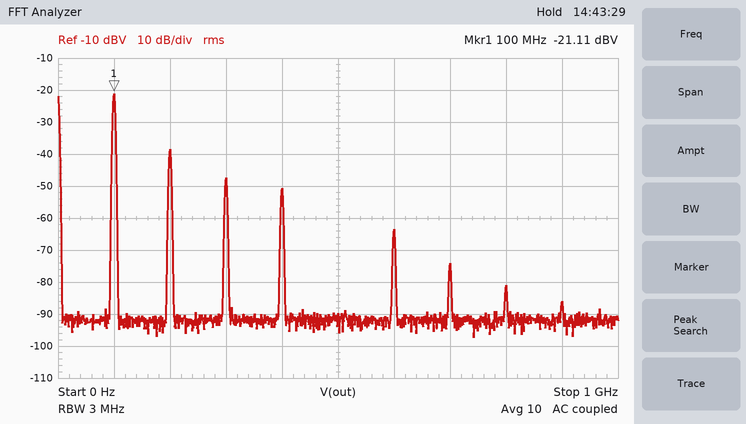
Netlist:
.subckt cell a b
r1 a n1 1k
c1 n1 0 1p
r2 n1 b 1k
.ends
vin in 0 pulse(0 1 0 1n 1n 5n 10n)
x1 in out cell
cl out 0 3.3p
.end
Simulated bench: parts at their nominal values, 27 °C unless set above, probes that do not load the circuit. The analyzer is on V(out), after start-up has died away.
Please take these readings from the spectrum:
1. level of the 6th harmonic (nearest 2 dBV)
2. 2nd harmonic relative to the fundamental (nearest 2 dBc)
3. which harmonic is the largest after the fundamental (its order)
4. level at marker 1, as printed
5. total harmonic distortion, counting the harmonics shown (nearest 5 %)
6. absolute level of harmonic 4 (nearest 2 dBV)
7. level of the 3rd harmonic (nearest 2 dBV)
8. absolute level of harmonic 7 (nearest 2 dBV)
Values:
-64 dBV
-18 dBc
2
-21.11 dBV
15 %
-50 dBV
-48 dBV
-74 dBV
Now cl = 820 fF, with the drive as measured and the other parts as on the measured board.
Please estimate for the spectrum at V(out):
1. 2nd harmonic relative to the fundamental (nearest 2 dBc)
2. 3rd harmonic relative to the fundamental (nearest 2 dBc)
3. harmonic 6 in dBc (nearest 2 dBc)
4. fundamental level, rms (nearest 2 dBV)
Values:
-16 dBc
-24 dBc
-40 dBc
-12 dBV
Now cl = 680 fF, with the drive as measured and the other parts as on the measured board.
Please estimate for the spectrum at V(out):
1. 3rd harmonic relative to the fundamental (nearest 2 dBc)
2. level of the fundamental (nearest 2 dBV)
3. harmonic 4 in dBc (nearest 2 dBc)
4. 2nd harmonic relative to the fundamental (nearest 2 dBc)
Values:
-24 dBc
-12 dBV
-26 dBc
-16 dBc
